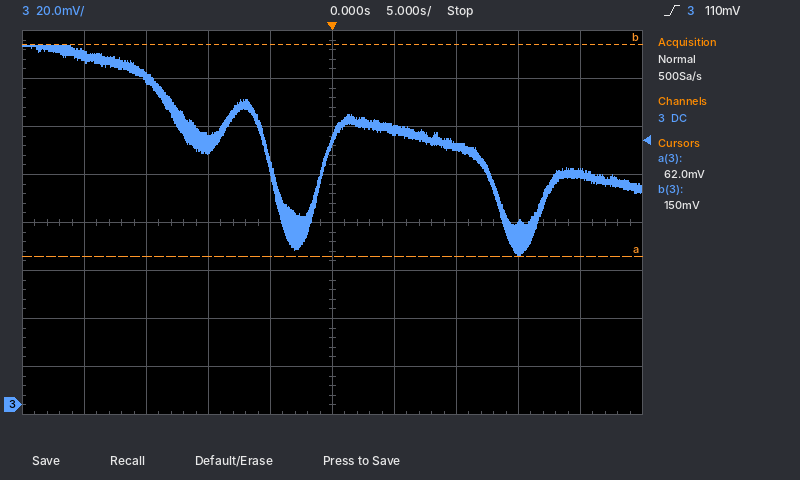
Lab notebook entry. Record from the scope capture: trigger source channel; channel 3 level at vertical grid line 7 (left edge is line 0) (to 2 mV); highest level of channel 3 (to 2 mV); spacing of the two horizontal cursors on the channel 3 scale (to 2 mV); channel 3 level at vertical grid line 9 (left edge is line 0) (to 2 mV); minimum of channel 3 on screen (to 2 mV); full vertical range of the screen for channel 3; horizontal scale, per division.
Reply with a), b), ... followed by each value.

a) channel 3
b) 108 mV
c) 150 mV
d) 88 mV
e) 96 mV
f) 62 mV
g) 160 mV
h) 5 s
